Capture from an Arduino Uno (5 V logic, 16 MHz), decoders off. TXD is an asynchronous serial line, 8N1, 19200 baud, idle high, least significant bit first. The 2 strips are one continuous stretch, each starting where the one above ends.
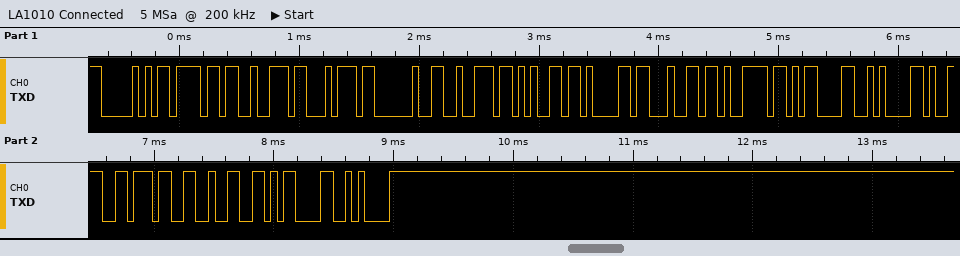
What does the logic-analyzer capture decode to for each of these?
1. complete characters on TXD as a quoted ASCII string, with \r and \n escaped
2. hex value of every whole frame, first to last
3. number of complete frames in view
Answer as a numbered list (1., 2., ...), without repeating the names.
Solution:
1. "Port ready\r\n972\r\n"
2. 50 6F 72 74 20 72 65 61 64 79 0D 0A 39 37 32 0D 0A
3. 17
